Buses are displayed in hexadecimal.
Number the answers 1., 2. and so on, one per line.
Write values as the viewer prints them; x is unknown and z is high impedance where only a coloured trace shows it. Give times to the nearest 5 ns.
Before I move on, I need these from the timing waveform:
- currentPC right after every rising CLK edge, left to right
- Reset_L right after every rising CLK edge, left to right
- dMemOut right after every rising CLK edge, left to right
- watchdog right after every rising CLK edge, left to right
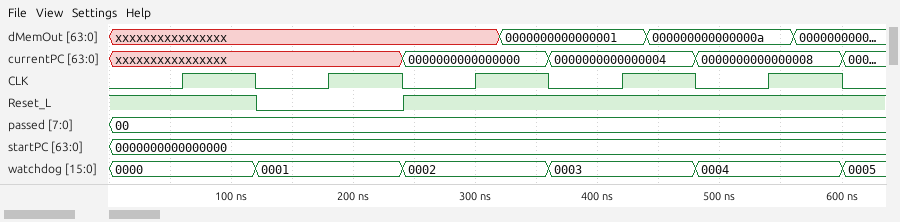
1. xxxxxxxxxxxxxxxx, xxxxxxxxxxxxxxxx, 0000000000000000, 0000000000000004, 0000000000000008
2. 1 0 1 1 1
3. xxxxxxxxxxxxxxxx, xxxxxxxxxxxxxxxx, xxxxxxxxxxxxxxxx, 0000000000000001, 000000000000000a
4. 0000, 0001, 0002, 0003, 0004
